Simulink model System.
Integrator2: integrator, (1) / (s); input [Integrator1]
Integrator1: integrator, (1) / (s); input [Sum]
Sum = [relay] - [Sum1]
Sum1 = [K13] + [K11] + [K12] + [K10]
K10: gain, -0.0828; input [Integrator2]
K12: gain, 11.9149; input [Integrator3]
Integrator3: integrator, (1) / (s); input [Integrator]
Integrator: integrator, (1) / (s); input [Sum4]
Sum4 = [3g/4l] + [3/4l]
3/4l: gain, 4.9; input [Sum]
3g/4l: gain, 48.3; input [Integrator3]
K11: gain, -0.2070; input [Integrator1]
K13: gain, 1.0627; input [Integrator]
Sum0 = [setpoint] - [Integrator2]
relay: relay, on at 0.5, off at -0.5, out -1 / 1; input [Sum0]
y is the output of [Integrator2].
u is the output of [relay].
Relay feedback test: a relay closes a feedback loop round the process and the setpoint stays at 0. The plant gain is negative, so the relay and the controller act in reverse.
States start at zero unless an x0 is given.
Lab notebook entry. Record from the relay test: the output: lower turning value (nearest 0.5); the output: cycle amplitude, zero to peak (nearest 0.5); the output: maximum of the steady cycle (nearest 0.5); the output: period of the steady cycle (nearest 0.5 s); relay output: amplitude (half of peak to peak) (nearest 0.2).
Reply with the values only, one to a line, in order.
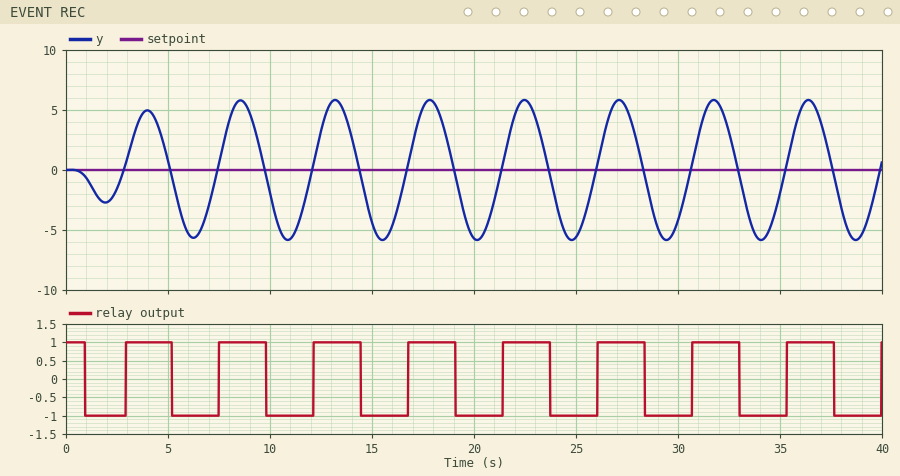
-6.0
6.0
6.0
4.5 s
1.0
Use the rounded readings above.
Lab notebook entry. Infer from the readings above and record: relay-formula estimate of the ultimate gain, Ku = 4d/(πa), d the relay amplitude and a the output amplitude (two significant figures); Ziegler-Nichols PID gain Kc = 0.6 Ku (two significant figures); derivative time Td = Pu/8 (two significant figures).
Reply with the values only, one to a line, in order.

0.21
0.13
0.56 s
